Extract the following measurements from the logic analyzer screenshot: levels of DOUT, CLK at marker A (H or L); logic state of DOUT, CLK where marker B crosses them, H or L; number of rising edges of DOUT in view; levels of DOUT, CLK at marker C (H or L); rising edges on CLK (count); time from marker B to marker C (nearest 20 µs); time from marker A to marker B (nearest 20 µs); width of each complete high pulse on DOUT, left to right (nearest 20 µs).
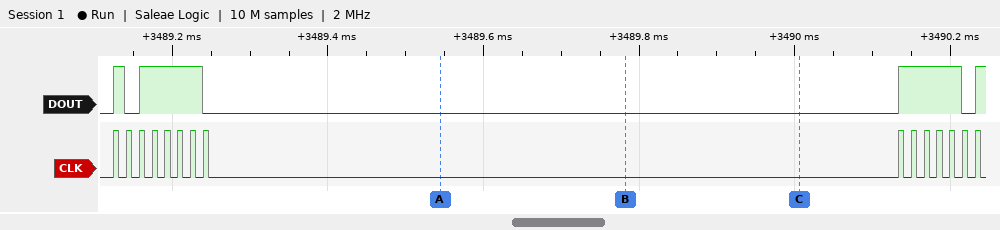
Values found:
DOUT=L, CLK=L
DOUT=L, CLK=L
4
DOUT=L, CLK=L
15
220 µs
240 µs
20 µs, 80 µs, 80 µs
